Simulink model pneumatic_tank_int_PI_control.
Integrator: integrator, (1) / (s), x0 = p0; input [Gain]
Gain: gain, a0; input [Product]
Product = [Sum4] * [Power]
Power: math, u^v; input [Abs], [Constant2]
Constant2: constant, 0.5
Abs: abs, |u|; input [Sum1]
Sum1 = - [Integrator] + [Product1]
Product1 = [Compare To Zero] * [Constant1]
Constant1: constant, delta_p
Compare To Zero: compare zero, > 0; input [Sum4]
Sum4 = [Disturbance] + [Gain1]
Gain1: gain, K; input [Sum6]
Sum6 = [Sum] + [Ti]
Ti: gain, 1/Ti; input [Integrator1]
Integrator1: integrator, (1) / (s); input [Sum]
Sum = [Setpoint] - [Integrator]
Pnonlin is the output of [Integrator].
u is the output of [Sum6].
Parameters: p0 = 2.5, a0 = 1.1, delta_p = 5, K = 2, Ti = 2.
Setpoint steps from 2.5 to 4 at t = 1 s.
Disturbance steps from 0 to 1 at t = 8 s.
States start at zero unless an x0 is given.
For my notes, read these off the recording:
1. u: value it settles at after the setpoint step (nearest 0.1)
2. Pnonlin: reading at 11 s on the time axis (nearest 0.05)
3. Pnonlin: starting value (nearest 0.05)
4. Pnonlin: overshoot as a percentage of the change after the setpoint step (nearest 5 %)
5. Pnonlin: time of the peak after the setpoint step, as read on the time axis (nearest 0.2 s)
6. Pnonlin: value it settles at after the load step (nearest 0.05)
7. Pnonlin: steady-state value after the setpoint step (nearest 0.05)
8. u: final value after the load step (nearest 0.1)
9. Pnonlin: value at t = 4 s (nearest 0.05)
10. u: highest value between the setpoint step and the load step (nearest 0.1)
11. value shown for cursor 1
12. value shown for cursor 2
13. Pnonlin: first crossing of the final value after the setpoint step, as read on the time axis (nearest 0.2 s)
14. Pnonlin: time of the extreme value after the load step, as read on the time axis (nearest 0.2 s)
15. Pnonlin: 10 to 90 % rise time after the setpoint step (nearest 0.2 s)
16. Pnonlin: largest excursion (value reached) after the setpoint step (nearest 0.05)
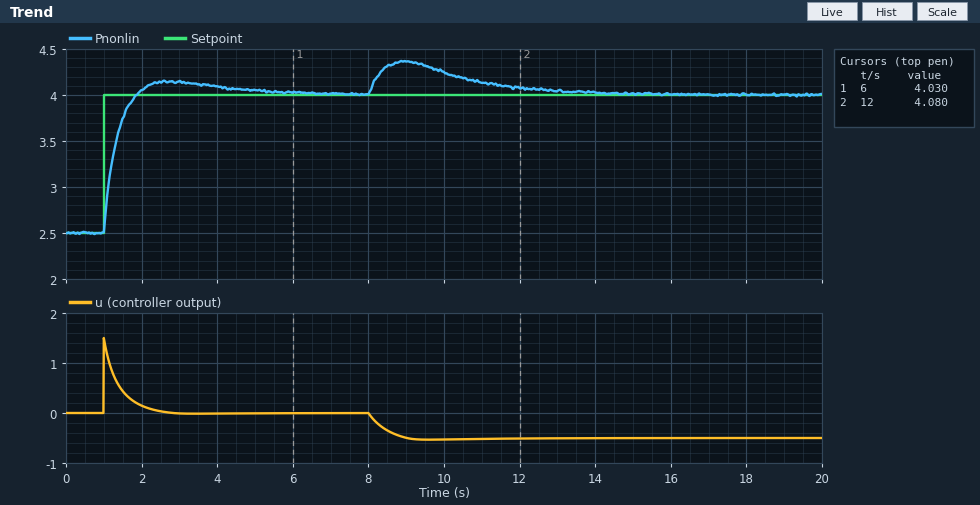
0.0
4.15
2.50
10 %
2.8 s
4.00
4.00
-0.5
4.10
1.5
4.030
4.080
1.8 s
9.0 s
0.6 s
4.15
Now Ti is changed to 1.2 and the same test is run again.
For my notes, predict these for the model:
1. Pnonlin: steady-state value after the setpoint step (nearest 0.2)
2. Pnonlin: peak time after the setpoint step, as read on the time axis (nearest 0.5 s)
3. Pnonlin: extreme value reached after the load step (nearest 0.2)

4.0
2.5 s
4.4
